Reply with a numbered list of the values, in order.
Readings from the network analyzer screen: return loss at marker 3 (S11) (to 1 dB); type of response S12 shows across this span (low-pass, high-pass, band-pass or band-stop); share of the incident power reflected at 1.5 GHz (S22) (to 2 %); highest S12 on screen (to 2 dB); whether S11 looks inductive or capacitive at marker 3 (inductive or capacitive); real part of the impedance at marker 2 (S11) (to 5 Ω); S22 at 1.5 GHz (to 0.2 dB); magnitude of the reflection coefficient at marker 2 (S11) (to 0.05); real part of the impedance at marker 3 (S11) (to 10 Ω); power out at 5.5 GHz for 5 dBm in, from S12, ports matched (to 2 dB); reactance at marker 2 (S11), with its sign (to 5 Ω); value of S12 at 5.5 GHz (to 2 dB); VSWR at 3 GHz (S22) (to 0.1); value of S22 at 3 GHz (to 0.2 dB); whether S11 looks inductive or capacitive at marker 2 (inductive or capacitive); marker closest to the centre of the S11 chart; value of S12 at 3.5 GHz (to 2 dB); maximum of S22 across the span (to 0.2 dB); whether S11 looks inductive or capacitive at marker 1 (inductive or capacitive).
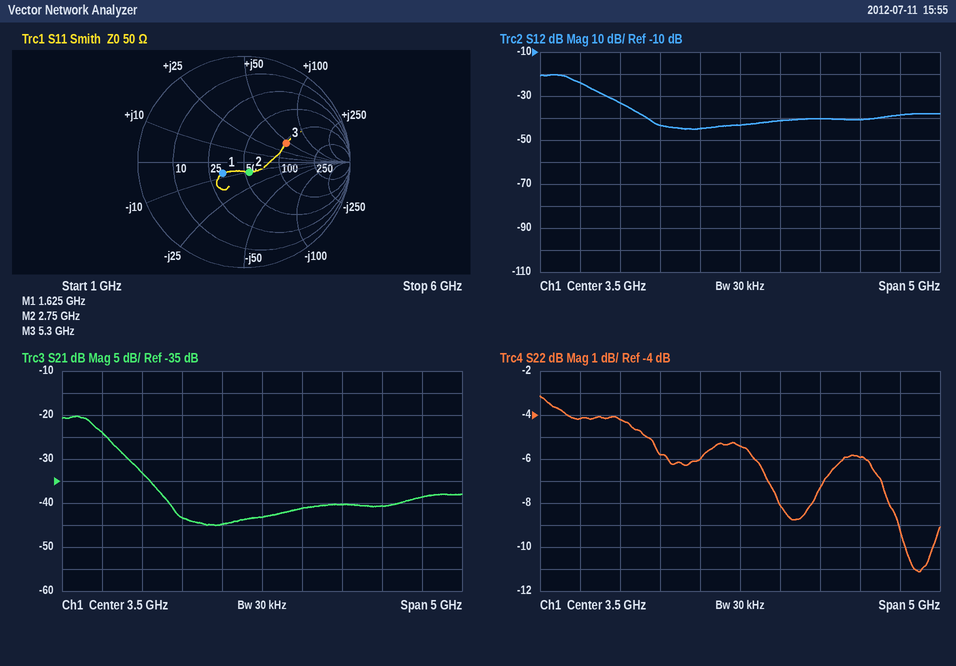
1. 7 dB
2. low-pass
3. 38 %
4. -20 dB
5. inductive
6. 55 Ω
7. -4.2 dB
8. 0.10
9. 100 Ω
10. -34 dBm
11. -10 Ω
12. -38 dB
13. 3.0
14. -6.0 dB
15. capacitive
16. marker 2
17. -44 dB
18. -3.2 dB
19. capacitive
